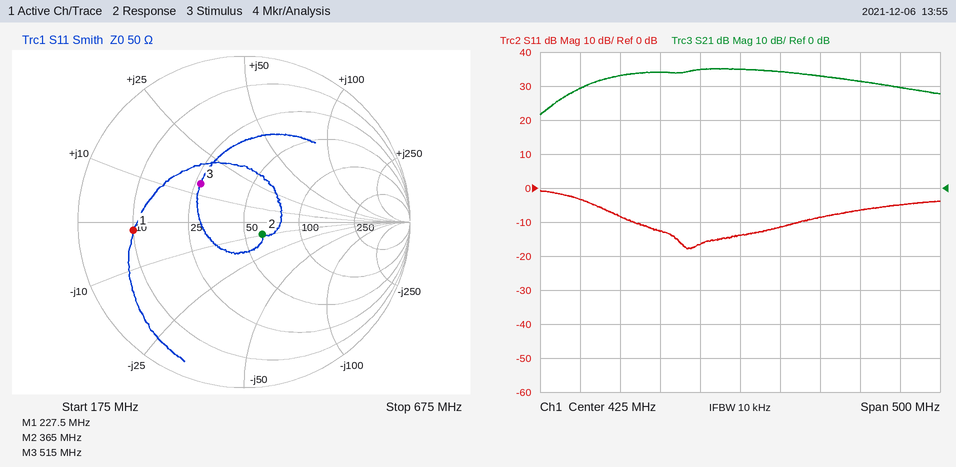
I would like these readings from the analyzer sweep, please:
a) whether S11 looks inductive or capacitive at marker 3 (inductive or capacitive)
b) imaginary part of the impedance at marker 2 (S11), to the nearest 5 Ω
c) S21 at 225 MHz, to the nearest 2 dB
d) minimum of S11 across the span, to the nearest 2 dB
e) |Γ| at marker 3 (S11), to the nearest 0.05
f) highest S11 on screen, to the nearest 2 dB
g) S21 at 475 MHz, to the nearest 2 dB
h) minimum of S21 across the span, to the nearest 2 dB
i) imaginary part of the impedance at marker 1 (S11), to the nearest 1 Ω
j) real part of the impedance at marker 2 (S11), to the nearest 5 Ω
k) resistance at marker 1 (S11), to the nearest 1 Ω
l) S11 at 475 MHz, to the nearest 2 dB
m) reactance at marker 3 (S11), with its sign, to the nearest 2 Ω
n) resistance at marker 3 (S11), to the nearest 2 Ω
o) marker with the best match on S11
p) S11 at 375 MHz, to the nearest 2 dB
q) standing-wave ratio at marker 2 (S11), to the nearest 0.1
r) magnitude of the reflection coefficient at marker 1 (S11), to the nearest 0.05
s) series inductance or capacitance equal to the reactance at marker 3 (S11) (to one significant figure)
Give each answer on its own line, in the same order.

inductive
-10 Ω
30 dB
-18 dB
0.35
0 dB
34 dB
22 dB
-2 Ω
60 Ω
10 Ω
-12 dB
+14 Ω
26 Ω
marker 2
-16 dB
1.3
0.65
4 nH
